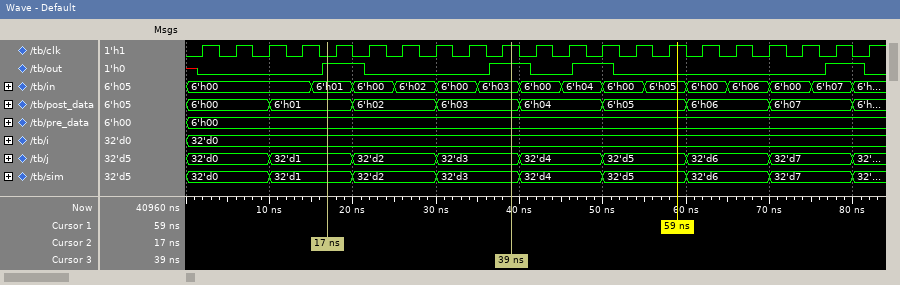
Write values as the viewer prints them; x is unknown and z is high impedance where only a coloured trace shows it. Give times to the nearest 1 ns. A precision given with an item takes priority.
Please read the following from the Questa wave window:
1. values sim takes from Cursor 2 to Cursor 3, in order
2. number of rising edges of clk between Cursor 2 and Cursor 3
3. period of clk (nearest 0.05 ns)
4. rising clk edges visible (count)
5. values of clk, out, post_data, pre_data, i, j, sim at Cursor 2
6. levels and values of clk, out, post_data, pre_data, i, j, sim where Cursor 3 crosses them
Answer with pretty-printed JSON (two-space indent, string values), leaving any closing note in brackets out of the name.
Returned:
{
  "values sim takes from Cursor 2 to Cursor 3, in order": "32'd1, 32'd2, 32'd3",
  "number of rising edges of clk between Cursor 2 and Cursor 3": "6",
  "period of clk": "4 ns",
  "rising clk edges visible": "21",
  "values of clk, out, post_data, pre_data, i, j, sim at Cursor 2": "clk=0, out=1, post_data=6'h01, pre_data=6'h00, i=32'd0, j=32'd1, sim=32'd1",
  "levels and values of clk, out, post_data, pre_data, i, j, sim where Cursor 3 crosses them": "clk=1, out=1, post_data=6'h03, pre_data=6'h00, i=32'd0, j=32'd3, sim=32'd3"
}
